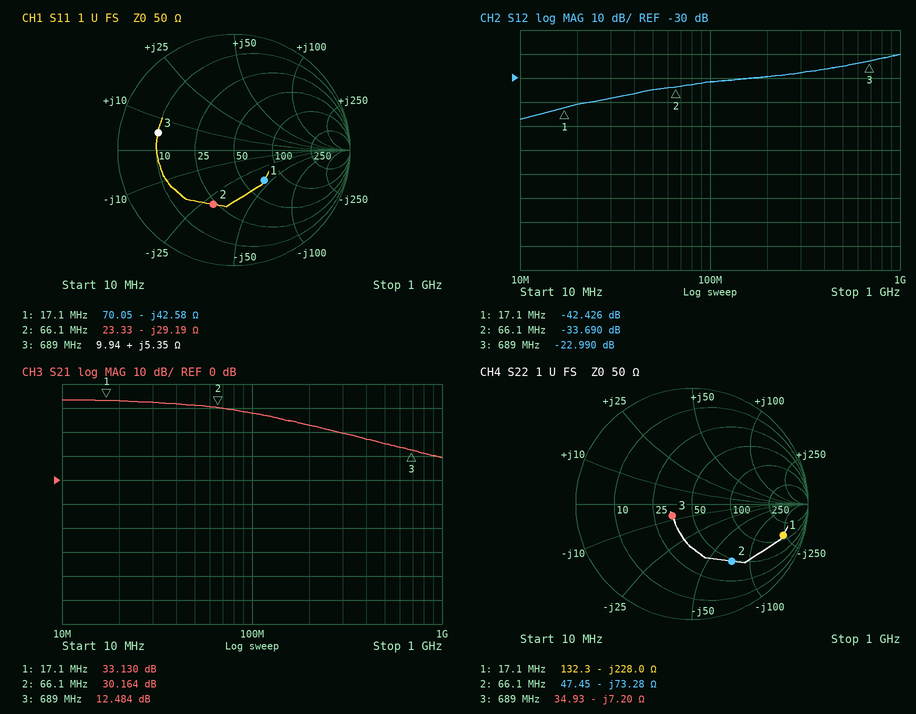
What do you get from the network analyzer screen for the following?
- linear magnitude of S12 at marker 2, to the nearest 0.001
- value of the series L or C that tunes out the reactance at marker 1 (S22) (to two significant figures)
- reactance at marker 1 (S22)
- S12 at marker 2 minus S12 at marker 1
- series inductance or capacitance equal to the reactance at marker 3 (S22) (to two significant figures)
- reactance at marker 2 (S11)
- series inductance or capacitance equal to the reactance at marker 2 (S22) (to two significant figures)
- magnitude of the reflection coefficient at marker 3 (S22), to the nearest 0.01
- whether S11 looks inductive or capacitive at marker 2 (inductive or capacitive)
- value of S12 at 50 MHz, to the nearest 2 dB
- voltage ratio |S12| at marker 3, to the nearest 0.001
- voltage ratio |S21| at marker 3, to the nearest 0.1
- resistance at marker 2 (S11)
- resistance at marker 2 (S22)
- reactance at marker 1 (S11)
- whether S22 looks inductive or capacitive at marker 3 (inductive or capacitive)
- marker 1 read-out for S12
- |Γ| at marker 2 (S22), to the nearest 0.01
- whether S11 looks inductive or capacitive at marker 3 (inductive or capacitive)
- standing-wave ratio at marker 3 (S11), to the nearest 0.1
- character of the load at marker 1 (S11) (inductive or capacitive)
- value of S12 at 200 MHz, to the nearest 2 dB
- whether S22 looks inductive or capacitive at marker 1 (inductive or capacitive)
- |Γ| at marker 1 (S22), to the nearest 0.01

0.021
2.1 µH
-228.0 Ω
8.736 dB
32 pF
-29.19 Ω
33 pF
0.20
capacitive
-34 dB
0.071
4.2
23.33 Ω
47.45 Ω
-42.58 Ω
capacitive
-42.426 dB
0.60
inductive
5.1
capacitive
-30 dB
capacitive
0.83
